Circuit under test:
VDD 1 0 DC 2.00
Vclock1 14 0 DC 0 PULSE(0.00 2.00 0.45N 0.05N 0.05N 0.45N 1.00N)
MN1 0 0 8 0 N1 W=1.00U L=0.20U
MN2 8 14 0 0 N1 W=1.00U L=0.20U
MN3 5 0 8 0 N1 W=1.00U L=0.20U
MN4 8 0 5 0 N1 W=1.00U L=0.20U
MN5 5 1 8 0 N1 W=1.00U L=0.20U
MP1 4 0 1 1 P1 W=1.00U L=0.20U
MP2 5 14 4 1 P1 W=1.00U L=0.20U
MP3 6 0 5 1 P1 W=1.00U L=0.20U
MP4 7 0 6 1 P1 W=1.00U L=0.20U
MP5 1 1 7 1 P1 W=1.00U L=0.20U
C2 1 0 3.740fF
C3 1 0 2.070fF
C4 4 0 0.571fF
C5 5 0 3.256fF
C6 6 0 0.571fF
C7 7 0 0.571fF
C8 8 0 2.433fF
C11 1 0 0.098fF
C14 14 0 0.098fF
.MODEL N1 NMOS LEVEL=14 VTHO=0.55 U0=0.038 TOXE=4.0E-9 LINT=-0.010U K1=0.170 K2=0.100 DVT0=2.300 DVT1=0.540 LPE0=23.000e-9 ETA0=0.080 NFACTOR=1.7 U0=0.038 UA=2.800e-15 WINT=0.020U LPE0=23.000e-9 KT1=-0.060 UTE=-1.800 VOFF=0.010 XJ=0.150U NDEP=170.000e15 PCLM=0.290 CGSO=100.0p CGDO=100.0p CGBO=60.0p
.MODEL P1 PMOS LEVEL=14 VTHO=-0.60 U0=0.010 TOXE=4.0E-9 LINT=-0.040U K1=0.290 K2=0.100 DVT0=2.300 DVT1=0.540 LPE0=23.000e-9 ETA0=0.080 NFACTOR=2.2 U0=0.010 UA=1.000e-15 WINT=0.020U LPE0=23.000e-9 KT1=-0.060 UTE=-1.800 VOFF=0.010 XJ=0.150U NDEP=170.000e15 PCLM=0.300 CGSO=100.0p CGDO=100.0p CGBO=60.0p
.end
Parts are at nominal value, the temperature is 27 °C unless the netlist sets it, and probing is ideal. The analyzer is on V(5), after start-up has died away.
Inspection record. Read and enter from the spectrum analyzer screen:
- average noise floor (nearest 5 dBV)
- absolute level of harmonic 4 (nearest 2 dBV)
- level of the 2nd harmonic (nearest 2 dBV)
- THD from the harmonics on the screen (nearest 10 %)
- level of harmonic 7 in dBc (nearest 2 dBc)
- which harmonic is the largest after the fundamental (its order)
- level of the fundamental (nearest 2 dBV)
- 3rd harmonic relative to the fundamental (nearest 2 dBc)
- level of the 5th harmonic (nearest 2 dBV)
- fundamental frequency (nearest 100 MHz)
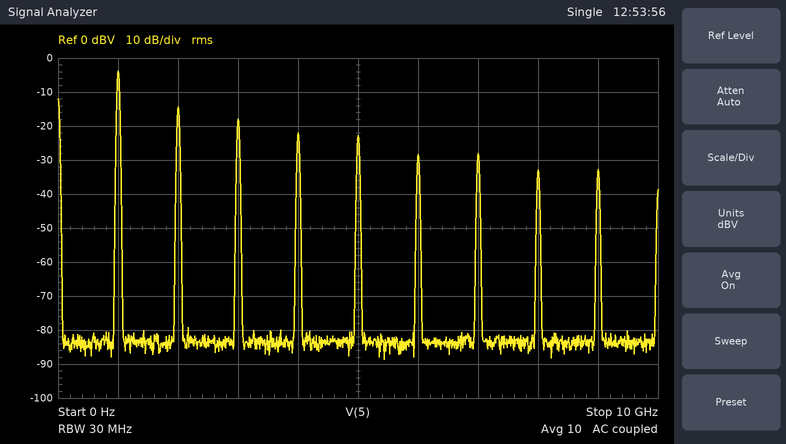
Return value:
-85 dBV
-22 dBV
-14 dBV
40 %
-24 dBc
2
-4 dBV
-14 dBc
-22 dBV
1.0 GHz
